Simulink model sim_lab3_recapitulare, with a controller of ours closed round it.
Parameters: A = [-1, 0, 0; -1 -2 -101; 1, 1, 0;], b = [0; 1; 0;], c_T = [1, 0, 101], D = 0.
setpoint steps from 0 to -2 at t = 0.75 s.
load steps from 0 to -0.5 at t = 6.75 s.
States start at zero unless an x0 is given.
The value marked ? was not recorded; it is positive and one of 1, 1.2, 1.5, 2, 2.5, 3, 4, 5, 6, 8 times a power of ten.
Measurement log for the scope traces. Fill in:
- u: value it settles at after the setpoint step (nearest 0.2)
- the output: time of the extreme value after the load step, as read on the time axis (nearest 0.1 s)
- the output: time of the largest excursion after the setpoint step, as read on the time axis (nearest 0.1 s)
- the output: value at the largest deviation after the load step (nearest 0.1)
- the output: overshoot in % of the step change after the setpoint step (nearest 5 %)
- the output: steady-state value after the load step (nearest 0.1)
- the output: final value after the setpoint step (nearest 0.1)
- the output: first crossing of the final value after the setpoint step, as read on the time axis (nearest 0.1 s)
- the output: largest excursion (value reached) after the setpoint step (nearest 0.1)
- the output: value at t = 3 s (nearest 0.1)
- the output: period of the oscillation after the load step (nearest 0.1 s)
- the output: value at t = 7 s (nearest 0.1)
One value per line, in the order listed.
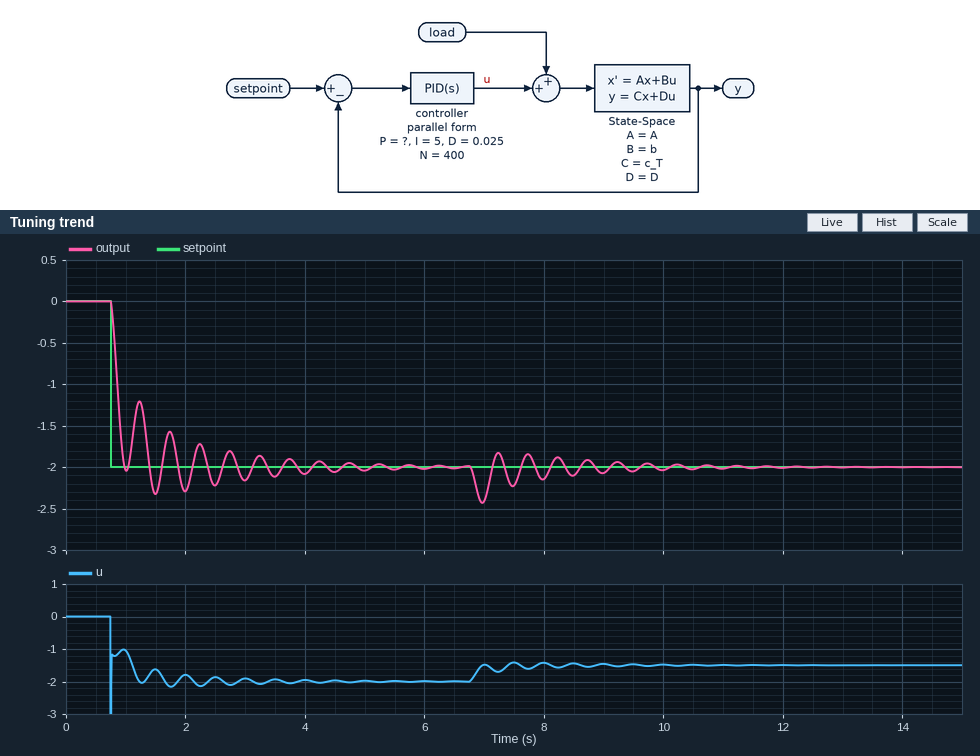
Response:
-2.0
7.0 s
1.5 s
-2.4
15 %
-2.0
-2.0
1.0 s
-2.3
-2.2
0.5 s
-2.4
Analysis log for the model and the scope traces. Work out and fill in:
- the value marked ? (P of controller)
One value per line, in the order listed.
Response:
0.6
